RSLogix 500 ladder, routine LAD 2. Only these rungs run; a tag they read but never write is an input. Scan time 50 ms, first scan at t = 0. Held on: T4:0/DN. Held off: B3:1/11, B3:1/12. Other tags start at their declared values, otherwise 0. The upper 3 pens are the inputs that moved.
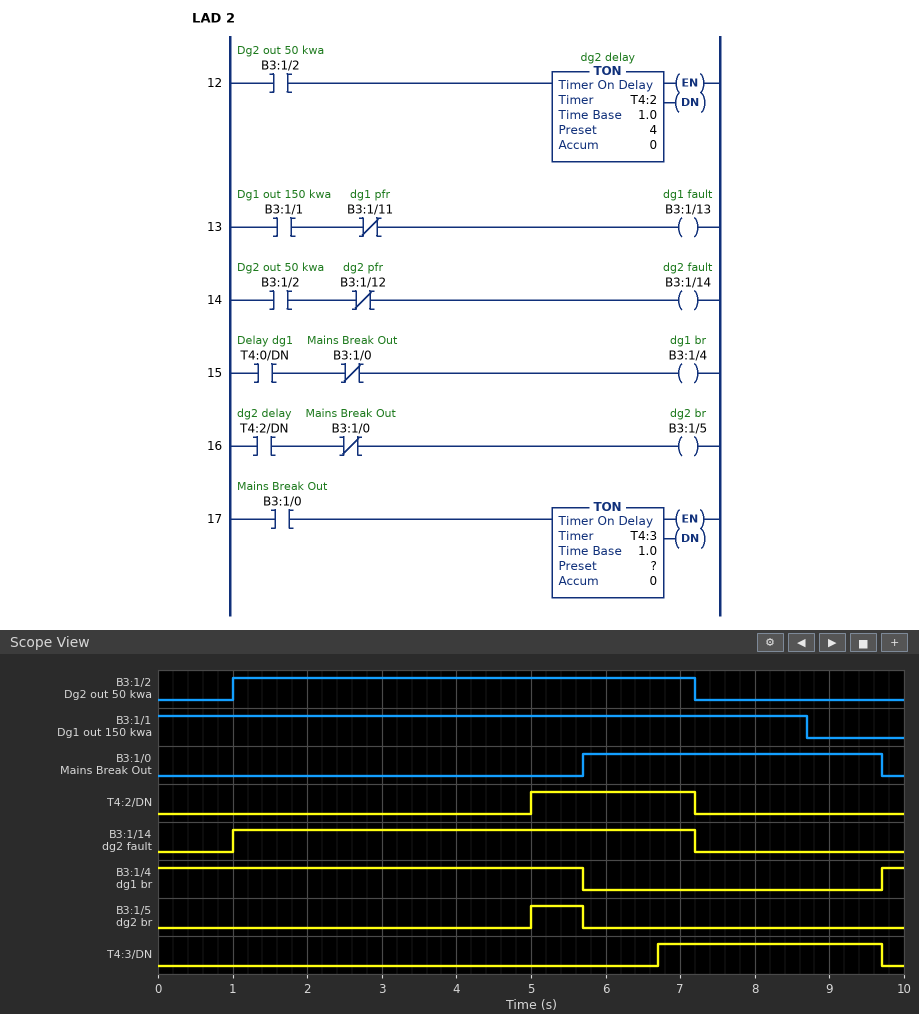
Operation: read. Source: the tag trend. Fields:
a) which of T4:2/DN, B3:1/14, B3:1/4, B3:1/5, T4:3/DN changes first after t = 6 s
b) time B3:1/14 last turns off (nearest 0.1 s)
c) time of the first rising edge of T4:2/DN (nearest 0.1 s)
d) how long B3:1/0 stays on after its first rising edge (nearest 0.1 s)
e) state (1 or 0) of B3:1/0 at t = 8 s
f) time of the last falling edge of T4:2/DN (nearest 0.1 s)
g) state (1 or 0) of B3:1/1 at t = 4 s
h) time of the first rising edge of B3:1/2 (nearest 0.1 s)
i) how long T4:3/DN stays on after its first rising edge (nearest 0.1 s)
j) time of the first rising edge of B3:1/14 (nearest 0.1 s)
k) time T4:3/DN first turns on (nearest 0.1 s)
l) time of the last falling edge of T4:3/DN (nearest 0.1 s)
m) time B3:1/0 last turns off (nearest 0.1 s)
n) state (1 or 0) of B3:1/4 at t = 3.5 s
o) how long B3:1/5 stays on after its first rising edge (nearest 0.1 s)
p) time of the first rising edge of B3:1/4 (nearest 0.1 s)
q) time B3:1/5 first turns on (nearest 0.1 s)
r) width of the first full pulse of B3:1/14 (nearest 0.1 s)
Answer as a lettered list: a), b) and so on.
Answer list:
a) T4:3/DN
b) 7.2 s
c) 5.0 s
d) 4.0 s
e) 1
f) 7.2 s
g) 1
h) 1.0 s
i) 3.0 s
j) 1.0 s
k) 6.7 s
l) 9.7 s
m) 9.7 s
n) 1
o) 0.7 s
p) 9.7 s
q) 5.0 s
r) 6.2 s
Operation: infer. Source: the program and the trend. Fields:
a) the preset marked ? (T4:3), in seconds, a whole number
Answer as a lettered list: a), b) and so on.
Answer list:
a) 1 s
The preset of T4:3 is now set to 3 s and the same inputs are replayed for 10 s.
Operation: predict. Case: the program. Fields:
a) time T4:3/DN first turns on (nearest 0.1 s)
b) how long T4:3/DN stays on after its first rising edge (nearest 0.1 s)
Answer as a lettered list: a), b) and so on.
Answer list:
a) 8.7 s
b) 1.0 s
